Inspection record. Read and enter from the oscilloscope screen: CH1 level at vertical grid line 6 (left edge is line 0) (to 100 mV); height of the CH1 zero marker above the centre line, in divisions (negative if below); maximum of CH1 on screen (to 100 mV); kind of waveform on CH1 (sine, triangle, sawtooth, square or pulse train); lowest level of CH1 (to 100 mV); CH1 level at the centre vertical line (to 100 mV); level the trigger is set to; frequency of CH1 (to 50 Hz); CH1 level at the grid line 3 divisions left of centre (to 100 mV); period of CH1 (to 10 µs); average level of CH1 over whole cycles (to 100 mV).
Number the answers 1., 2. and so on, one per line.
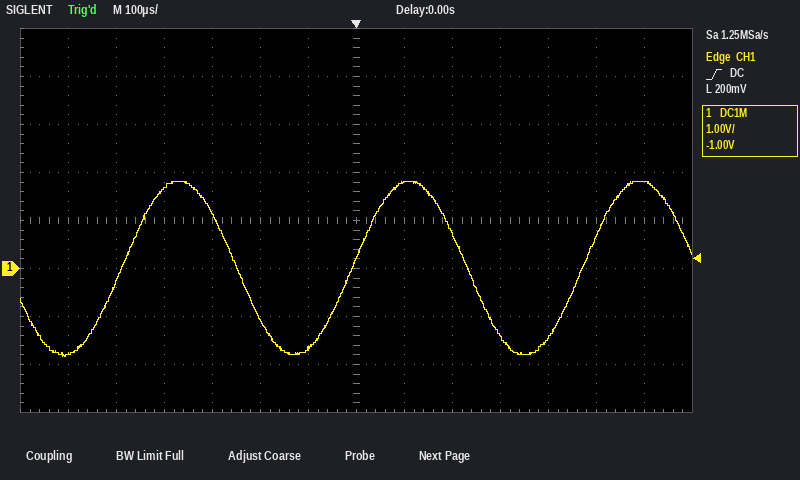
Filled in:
1. -1.7 V
2. -1.0 div
3. 1.8 V
4. sine
5. -1.8 V
6. 200 mV
7. 200 mV
8. 2.10 kHz
9. 1.1 V
10. 480 µs
11. 0.0 V
